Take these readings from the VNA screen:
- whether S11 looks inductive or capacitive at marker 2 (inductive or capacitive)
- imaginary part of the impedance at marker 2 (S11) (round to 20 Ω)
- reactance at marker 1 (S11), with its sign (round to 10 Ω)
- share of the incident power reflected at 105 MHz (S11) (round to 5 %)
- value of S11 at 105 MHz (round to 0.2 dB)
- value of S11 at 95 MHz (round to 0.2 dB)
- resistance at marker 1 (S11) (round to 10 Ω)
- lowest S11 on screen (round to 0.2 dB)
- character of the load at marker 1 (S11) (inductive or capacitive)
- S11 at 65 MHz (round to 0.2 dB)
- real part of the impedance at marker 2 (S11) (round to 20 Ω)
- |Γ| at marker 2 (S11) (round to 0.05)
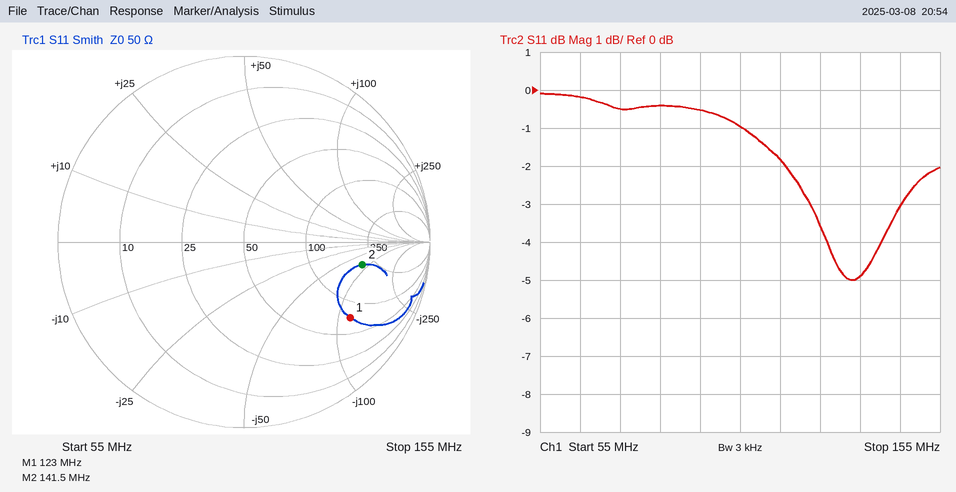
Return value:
capacitive
-80 Ω
-120 Ω
80 %
-1.0 dB
-0.6 dB
70 Ω
-5.0 dB
capacitive
-0.2 dB
200 Ω
0.65
